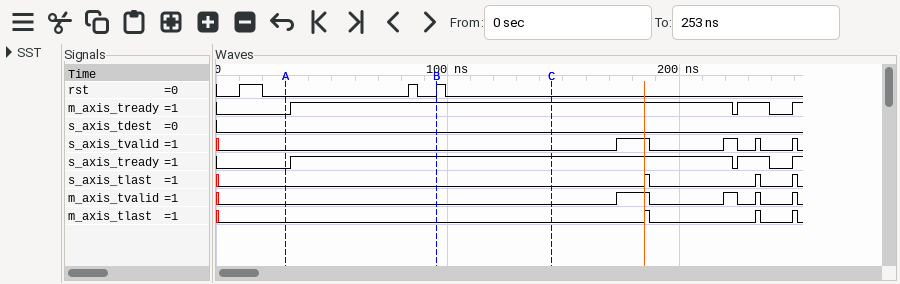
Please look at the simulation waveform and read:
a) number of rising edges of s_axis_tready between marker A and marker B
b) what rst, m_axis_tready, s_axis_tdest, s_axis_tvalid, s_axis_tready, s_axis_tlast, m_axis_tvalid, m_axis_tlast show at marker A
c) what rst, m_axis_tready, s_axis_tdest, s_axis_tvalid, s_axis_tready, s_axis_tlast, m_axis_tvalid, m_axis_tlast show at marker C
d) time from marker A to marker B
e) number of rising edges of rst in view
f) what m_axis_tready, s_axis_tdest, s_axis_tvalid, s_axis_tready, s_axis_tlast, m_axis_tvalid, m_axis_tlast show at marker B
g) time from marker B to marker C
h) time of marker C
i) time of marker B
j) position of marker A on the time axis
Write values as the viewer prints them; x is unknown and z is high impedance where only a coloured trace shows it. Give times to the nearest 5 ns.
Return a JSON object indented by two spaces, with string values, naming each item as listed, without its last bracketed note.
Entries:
{
  "number of rising edges of s_axis_tready between marker A and marker B": "1",
  "what rst, m_axis_tready, s_axis_tdest, s_axis_tvalid, s_axis_tready, s_axis_tlast, m_axis_tvalid, m_axis_tlast show at marker A": "rst=0, m_axis_tready=0, s_axis_tdest=0, s_axis_tvalid=0, s_axis_tready=0, s_axis_tlast=0, m_axis_tvalid=0, m_axis_tlast=0",
  "what rst, m_axis_tready, s_axis_tdest, s_axis_tvalid, s_axis_tready, s_axis_tlast, m_axis_tvalid, m_axis_tlast show at marker C": "rst=0, m_axis_tready=1, s_axis_tdest=0, s_axis_tvalid=0, s_axis_tready=1, s_axis_tlast=0, m_axis_tvalid=0, m_axis_tlast=0",
  "time from marker A to marker B": "65 ns",
  "number of rising edges of rst in view": "3",
  "what m_axis_tready, s_axis_tdest, s_axis_tvalid, s_axis_tready, s_axis_tlast, m_axis_tvalid, m_axis_tlast show at marker B": "m_axis_tready=1, s_axis_tdest=0, s_axis_tvalid=0, s_axis_tready=1, s_axis_tlast=0, m_axis_tvalid=0, m_axis_tlast=0",
  "time from marker B to marker C": "50 ns",
  "time of marker C": "145 ns",
  "time of marker B": "95 ns",
  "position of marker A on the time axis": "30 ns"
}
